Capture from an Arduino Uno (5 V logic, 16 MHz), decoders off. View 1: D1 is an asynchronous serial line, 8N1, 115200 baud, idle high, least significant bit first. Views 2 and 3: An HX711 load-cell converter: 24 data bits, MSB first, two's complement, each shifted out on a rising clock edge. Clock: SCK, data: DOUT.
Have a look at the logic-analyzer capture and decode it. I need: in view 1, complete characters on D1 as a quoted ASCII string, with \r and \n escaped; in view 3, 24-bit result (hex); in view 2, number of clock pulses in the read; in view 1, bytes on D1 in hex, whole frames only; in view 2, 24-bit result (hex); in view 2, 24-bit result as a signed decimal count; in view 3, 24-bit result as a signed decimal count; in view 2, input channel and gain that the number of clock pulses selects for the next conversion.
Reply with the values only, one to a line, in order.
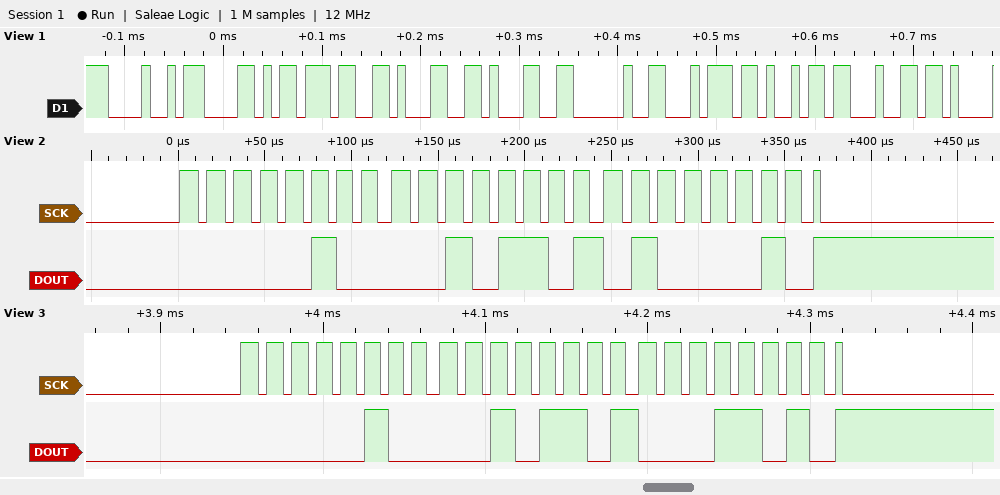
"HX711 tid"
0x042D1A
25
48 58 37 31 31 20 74 69 64
0x042D42
273730
273690
channel A, gain 128
